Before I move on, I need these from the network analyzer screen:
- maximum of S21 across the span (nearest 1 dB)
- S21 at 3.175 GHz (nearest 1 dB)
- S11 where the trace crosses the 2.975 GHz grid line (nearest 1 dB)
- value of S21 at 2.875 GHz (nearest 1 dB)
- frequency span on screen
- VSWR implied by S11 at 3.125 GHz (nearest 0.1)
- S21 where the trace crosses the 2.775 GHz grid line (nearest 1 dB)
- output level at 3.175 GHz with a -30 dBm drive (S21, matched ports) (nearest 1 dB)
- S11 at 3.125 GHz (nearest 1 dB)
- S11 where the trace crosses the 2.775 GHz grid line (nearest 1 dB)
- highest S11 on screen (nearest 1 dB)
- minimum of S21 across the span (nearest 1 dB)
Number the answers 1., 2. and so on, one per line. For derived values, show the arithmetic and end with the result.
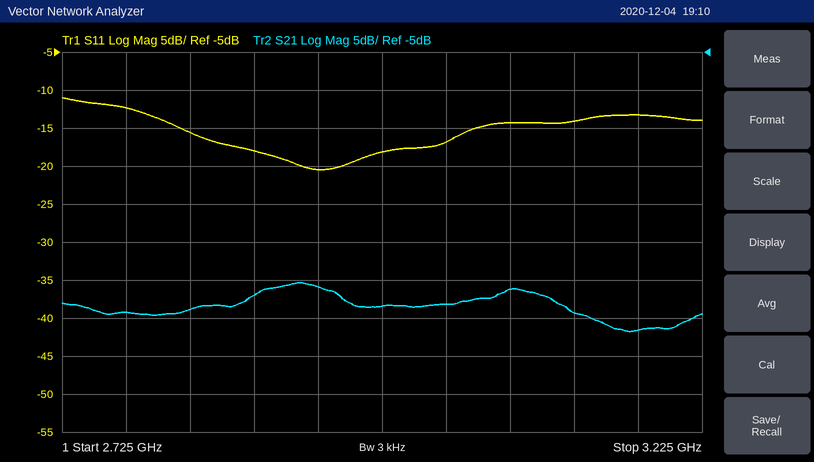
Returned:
1. -35 dB
2. -42 dB
3. -18 dB
4. -37 dB
5. 500 MHz
6. |Γ| = 10^(-14/20) = 0.1995; VSWR = (1 + 0.1995)/(1 − 0.1995) ≈ 1.5
7. -39 dB
8. -30 dBm + (-42 dB) = -72 dBm
9. -14 dB
10. -12 dB
11. -11 dB
12. -42 dB
